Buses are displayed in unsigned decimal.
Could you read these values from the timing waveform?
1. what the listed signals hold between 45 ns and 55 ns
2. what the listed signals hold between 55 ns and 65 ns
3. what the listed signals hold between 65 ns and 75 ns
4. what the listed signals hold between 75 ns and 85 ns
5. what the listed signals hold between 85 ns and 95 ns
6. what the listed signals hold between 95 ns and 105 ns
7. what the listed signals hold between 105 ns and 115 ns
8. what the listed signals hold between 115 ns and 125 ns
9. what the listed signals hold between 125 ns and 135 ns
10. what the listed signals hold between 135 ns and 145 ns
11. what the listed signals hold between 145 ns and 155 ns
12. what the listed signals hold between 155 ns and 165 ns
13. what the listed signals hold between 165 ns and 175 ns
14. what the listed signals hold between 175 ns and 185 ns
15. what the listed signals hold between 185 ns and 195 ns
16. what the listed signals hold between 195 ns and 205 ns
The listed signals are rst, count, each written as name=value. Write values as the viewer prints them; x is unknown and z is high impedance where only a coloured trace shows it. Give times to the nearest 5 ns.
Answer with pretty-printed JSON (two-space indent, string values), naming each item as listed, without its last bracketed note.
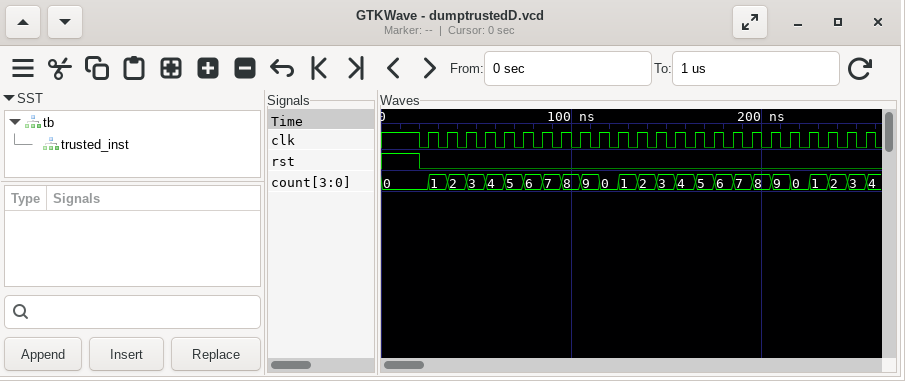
{
  "what the listed signals hold between 45 ns and 55 ns": "rst=0, count=3",
  "what the listed signals hold between 55 ns and 65 ns": "rst=0, count=4",
  "what the listed signals hold between 65 ns and 75 ns": "rst=0, count=5",
  "what the listed signals hold between 75 ns and 85 ns": "rst=0, count=6",
  "what the listed signals hold between 85 ns and 95 ns": "rst=0, count=7",
  "what the listed signals hold between 95 ns and 105 ns": "rst=0, count=8",
  "what the listed signals hold between 105 ns and 115 ns": "rst=0, count=9",
  "what the listed signals hold between 115 ns and 125 ns": "rst=0, count=0",
  "what the listed signals hold between 125 ns and 135 ns": "rst=0, count=1",
  "what the listed signals hold between 135 ns and 145 ns": "rst=0, count=2",
  "what the listed signals hold between 145 ns and 155 ns": "rst=0, count=3",
  "what the listed signals hold between 155 ns and 165 ns": "rst=0, count=4",
  "what the listed signals hold between 165 ns and 175 ns": "rst=0, count=5",
  "what the listed signals hold between 175 ns and 185 ns": "rst=0, count=6",
  "what the listed signals hold between 185 ns and 195 ns": "rst=0, count=7",
  "what the listed signals hold between 195 ns and 205 ns": "rst=0, count=8"
}
